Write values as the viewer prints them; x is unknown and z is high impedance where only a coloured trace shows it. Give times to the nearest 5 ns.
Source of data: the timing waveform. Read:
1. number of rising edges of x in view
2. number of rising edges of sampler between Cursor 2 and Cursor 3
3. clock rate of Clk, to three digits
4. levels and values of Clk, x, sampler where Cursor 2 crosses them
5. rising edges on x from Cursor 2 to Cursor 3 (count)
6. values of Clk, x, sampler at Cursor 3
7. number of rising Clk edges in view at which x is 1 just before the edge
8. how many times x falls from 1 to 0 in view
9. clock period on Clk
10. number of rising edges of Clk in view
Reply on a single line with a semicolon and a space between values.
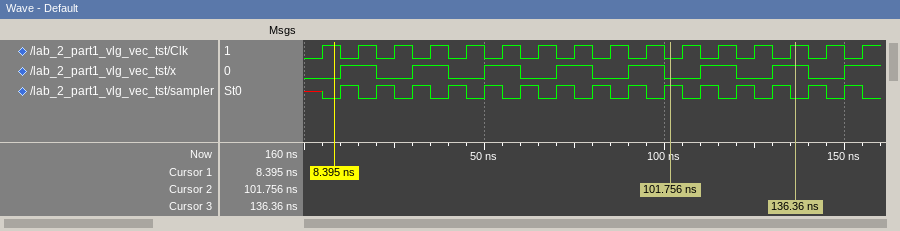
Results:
8; 3; 100 MHz; Clk=0, x=0, sampler=1; 2; Clk=1, x=1, sampler=0; 8; 7; 10 ns; 16
